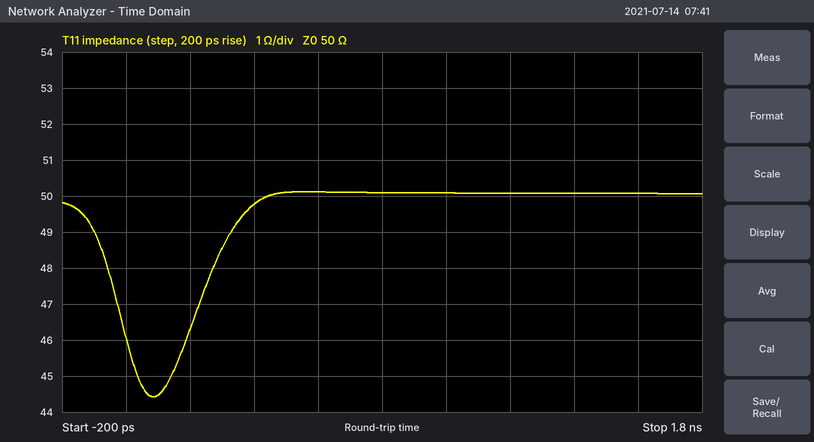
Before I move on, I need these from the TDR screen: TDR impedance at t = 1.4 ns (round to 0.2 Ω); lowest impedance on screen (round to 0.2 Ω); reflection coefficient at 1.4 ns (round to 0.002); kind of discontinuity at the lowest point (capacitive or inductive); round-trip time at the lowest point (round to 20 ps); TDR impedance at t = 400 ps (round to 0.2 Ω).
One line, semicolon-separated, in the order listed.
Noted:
50.0 Ω; 44.4 Ω; 0.000; capacitive; 80 ps; 49.8 Ω
